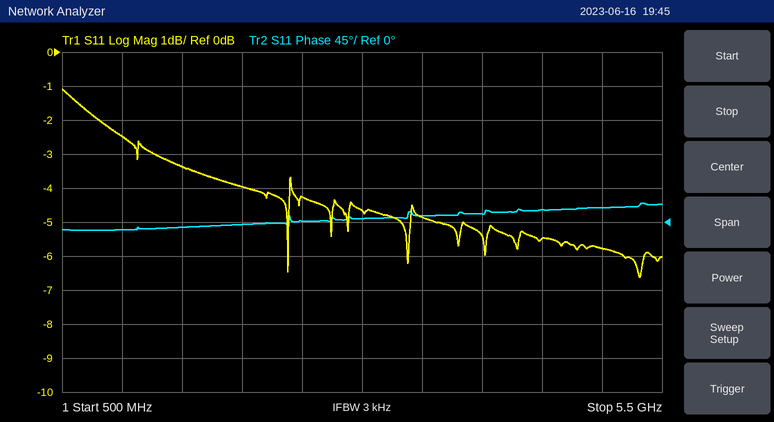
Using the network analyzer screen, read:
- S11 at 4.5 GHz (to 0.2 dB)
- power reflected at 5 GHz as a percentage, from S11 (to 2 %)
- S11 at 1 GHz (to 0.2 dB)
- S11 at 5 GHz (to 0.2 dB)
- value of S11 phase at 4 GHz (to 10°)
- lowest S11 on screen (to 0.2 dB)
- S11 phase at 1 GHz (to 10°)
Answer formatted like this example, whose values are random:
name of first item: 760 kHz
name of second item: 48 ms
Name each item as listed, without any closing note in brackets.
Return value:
S11 at 4.5 GHz: -5.4 dB
power reflected at 5 GHz as a percentage, from S11: 26 %
S11 at 1 GHz: -2.4 dB
S11 at 5 GHz: -5.8 dB
value of S11 phase at 4 GHz: 10°
lowest S11 on screen: -6.6 dB
S11 phase at 1 GHz: -10°
